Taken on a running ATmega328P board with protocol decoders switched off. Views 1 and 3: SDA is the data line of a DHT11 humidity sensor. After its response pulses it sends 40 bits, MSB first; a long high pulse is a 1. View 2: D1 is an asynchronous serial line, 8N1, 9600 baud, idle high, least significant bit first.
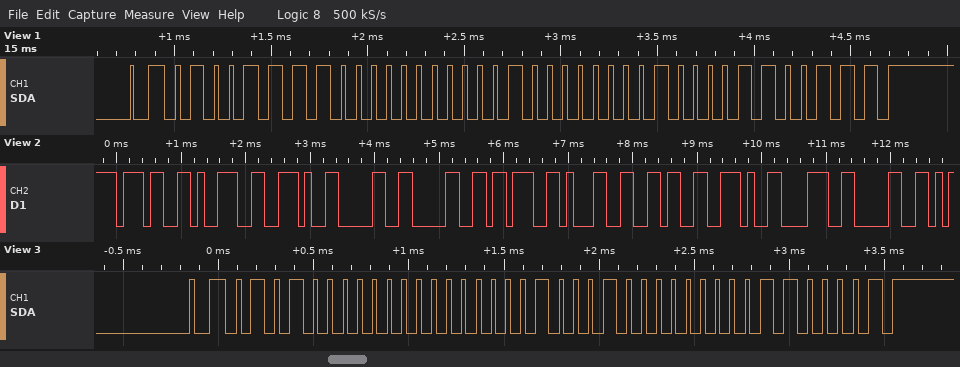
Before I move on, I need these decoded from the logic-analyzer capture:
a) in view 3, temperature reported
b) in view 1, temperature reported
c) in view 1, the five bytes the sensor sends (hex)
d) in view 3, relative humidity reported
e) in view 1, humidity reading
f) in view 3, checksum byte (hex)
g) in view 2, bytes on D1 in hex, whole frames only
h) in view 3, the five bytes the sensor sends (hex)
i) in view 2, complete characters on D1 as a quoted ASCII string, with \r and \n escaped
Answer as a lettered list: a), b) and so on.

a) 17.0 °C
b) 16.8 °C
c) 4F 00 10 08 67
d) 80 %
e) 79 %
f) 0x61
g) 37 39 2E 30 30 3B 31 36 2E 38 30
h) 50 00 11 00 61
i) "79.00;16.80"
